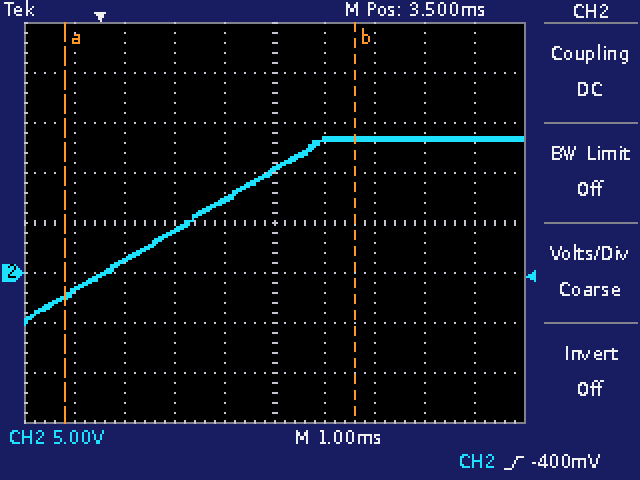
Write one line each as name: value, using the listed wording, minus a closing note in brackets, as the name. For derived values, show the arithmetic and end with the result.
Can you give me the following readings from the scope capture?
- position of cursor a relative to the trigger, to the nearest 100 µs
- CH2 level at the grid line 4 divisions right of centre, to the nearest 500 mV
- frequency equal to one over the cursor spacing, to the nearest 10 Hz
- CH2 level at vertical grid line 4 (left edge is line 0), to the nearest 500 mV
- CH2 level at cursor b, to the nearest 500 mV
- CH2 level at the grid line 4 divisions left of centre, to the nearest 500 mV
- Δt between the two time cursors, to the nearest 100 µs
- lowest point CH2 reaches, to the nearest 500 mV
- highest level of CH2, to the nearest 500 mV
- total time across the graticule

position of cursor a relative to the trigger, to the nearest 100 µs: -700 µs
CH2 level at the grid line 4 divisions right of centre, to the nearest 500 mV: 13.5 V
frequency equal to one over the cursor spacing, to the nearest 10 Hz: 1 / 5.8 ms ≈ 170 Hz
CH2 level at vertical grid line 4 (left edge is line 0), to the nearest 500 mV: 7.0 V
CH2 level at cursor b, to the nearest 500 mV: 13.5 V
CH2 level at the grid line 4 divisions left of centre, to the nearest 500 mV: -2.0 V
Δt between the two time cursors, to the nearest 100 µs: 5.8 ms
lowest point CH2 reaches, to the nearest 500 mV: -5.0 V
highest level of CH2, to the nearest 500 mV: 13.5 V
total time across the graticule: 10 ms
